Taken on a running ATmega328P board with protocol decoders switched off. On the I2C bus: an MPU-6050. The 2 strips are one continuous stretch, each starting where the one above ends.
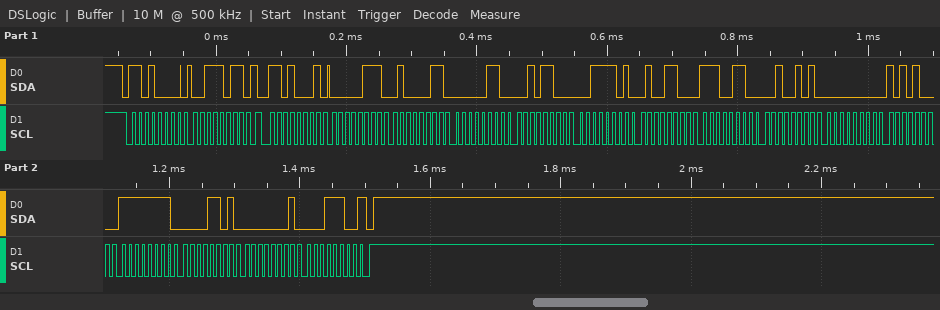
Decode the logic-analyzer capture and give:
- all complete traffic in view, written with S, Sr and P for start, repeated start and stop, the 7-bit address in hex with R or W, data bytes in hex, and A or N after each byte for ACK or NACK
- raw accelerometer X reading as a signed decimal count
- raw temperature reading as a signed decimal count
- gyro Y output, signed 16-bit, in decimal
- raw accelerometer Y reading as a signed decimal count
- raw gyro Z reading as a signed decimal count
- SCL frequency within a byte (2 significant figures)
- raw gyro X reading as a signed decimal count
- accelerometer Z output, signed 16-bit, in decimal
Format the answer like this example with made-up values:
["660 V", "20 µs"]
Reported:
["S 68W A 3B A Sr 68R A 07 A 43 A 06 A 2C A 3D A 4C A E6 A 25 A 00 A A8 A FF A 0D A 01 A 1C N P", "1859", "-6619", "-243", "1580", "284", "100 kHz", "168", "15692"]
